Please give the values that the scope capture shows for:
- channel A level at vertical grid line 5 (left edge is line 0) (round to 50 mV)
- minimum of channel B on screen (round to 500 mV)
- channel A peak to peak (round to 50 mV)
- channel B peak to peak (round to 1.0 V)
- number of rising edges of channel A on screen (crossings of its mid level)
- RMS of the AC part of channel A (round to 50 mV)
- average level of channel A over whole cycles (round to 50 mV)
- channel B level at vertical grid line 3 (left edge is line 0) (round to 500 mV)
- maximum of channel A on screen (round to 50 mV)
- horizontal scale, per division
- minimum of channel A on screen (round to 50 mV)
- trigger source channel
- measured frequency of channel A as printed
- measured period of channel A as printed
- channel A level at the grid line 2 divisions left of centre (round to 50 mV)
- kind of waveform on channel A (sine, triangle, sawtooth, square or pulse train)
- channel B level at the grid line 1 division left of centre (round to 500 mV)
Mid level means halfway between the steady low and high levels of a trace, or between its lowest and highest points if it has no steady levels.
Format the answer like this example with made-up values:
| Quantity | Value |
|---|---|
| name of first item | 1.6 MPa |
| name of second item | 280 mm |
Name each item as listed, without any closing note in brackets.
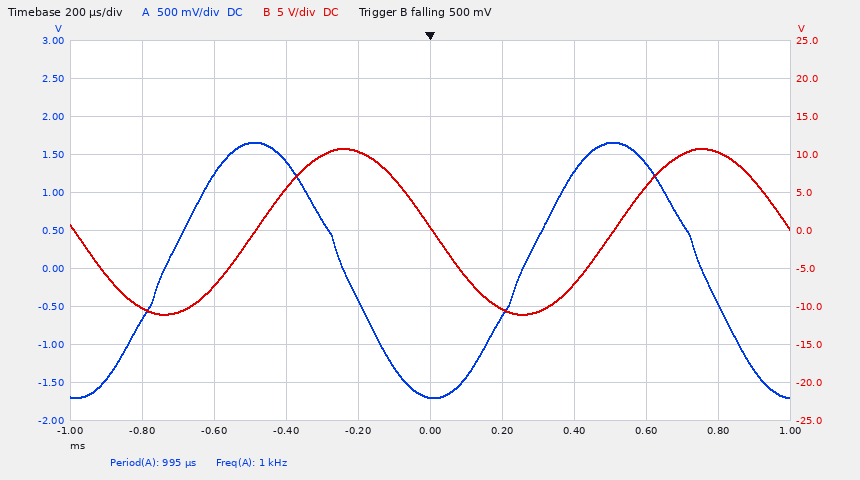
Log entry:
| Quantity | Value |
|---|---|
| channel A level at vertical grid line 5 (left edge is line 0) | -1.70 V |
| minimum of channel B on screen | -11.0 V |
| channel A peak to peak | 3.35 V |
| channel B peak to peak | 22.0 V |
| number of rising edges of channel A on screen | 2 |
| RMS of the AC part of channel A | 1.20 V |
| average level of channel A over whole cycles | 0 mV |
| channel B level at vertical grid line 3 (left edge is line 0) | 5.5 V |
| maximum of channel A on screen | 1.65 V |
| horizontal scale, per division | 200 µs |
| minimum of channel A on screen | -1.70 V |
| trigger source channel | channel B |
| measured frequency of channel A as printed | 1 kHz |
| measured period of channel A as printed | 995 µs |
| channel A level at the grid line 2 divisions left of centre | 1.40 V |
| kind of waveform on channel A | sine |
| channel B level at the grid line 1 division left of centre | 10.5 V |
